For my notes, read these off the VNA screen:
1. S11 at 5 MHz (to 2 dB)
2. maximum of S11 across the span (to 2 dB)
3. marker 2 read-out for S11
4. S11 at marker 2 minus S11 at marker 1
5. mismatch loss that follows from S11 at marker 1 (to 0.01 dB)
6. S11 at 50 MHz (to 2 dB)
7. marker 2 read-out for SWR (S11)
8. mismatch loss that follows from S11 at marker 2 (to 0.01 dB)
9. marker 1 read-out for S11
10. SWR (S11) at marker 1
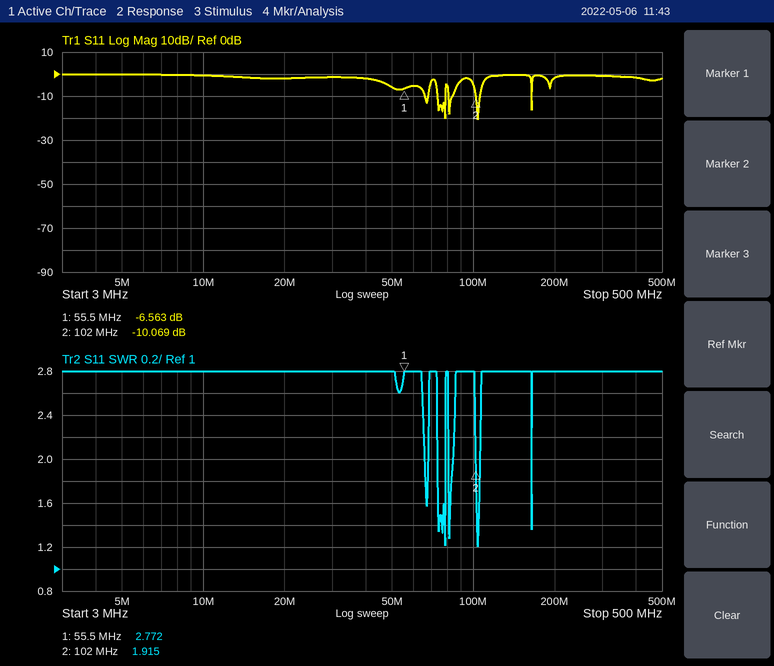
0 dB
0 dB
-10.069 dB
-3.506 dB
1.08 dB
-6 dB
1.915
0.45 dB
-6.563 dB
2.772
